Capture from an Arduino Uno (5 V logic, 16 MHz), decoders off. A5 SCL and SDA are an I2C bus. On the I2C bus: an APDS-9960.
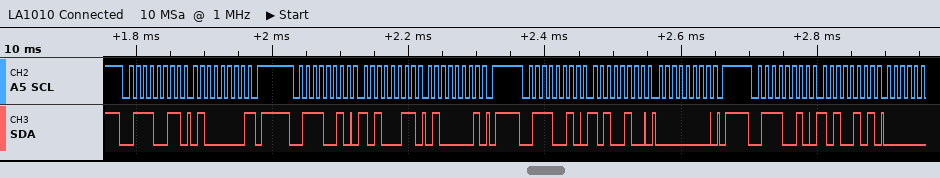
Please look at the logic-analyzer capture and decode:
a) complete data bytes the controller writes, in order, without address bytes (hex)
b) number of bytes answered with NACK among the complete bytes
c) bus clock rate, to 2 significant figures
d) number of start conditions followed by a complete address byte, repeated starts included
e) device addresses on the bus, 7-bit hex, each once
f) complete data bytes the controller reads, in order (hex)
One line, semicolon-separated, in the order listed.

A3 41 A4 00 A5; 1; 100 kHz; 4; 0x39; 40
